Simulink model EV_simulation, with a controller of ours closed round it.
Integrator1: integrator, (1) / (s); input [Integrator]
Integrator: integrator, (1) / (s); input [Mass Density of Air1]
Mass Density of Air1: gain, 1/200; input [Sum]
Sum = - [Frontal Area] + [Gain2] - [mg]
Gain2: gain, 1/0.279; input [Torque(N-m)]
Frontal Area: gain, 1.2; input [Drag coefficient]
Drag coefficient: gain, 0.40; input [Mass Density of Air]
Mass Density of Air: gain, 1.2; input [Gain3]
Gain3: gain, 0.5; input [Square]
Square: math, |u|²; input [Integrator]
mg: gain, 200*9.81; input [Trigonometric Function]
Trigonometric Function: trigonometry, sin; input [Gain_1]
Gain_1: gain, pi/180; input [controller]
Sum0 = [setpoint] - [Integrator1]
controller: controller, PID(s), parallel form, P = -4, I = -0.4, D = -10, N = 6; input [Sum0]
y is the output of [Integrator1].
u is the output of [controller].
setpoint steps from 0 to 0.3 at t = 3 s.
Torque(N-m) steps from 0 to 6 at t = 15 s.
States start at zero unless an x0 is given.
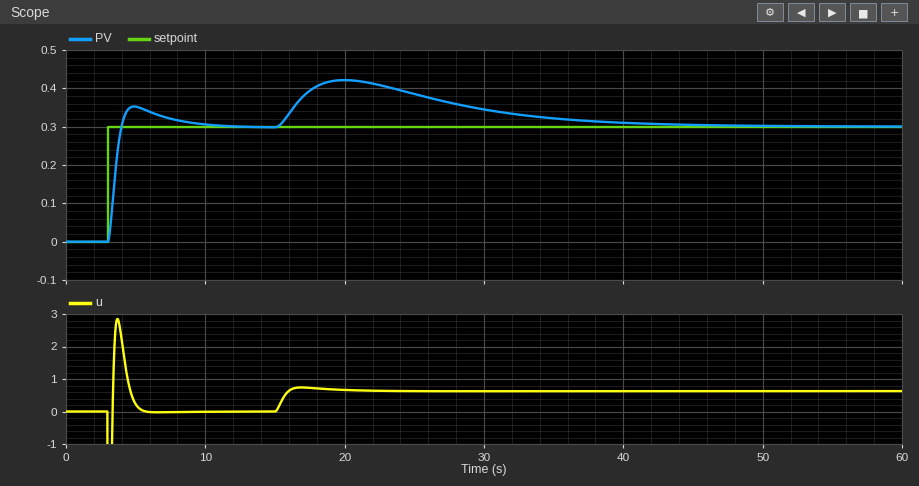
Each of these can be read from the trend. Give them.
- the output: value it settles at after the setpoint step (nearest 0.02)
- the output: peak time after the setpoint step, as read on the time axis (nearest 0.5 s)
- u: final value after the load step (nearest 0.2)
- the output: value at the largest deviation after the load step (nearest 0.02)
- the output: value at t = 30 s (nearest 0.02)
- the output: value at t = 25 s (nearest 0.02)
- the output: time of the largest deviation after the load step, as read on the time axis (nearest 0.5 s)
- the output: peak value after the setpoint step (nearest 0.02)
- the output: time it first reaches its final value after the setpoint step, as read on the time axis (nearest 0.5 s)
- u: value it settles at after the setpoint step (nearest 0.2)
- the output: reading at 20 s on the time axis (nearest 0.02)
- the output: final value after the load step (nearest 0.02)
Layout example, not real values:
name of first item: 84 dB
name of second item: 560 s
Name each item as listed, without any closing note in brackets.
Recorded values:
the output: value it settles at after the setpoint step: 0.30
the output: peak time after the setpoint step, as read on the time axis: 5.0 s
u: final value after the load step: 0.6
the output: value at the largest deviation after the load step: 0.42
the output: value at t = 30 s: 0.34
the output: value at t = 25 s: 0.38
the output: time of the largest deviation after the load step, as read on the time axis: 20.0 s
the output: peak value after the setpoint step: 0.36
the output: time it first reaches its final value after the setpoint step, as read on the time axis: 4.0 s
u: value it settles at after the setpoint step: 0.0
the output: reading at 20 s on the time axis: 0.42
the output: final value after the load step: 0.30
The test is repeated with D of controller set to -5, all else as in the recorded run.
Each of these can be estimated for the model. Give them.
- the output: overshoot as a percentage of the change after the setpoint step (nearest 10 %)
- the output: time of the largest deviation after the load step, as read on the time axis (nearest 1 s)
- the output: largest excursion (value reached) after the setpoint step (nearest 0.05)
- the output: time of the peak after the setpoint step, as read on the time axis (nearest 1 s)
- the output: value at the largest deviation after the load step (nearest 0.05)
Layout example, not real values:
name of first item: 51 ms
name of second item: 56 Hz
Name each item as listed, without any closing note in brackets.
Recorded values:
the output: overshoot as a percentage of the change after the setpoint step: 40 %
the output: time of the largest deviation after the load step, as read on the time axis: 19 s
the output: largest excursion (value reached) after the setpoint step: 0.40
the output: time of the peak after the setpoint step, as read on the time axis: 6 s
the output: value at the largest deviation after the load step: 0.45
